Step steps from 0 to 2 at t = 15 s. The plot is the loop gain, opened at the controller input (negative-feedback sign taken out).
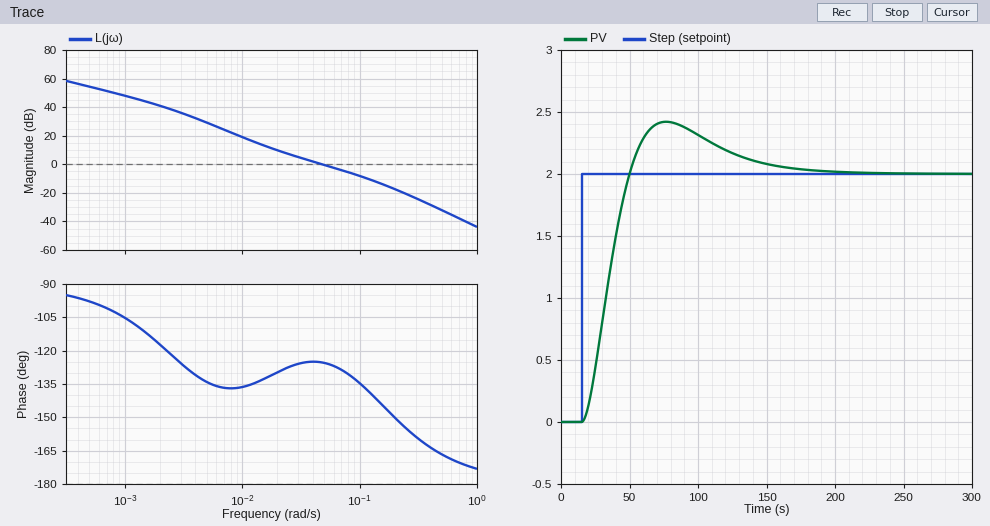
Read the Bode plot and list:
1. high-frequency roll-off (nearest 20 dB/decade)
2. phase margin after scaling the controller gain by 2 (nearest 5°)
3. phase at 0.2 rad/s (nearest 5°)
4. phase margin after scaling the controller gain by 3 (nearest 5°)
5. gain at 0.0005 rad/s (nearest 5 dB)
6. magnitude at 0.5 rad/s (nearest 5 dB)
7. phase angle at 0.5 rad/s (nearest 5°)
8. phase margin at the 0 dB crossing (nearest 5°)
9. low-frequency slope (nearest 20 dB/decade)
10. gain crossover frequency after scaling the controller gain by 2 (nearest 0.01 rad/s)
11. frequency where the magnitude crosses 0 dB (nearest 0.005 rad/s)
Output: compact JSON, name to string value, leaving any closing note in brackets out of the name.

{"high-frequency roll-off": "-40 dB/decade", "phase margin after scaling the controller gain by 2": "50°", "phase at 0.2 rad/s": "-150°", "phase margin after scaling the controller gain by 3": "45°", "gain at 0.0005 rad/s": "55 dB", "magnitude at 0.5 rad/s": "-30 dB", "phase angle at 0.5 rad/s": "-165°", "phase margin at the 0 dB crossing": "55°", "low-frequency slope": "-20 dB/decade", "gain crossover frequency after scaling the controller gain by 2": "0.08 rad/s", "frequency where the magnitude crosses 0 dB": "0.050 rad/s"}
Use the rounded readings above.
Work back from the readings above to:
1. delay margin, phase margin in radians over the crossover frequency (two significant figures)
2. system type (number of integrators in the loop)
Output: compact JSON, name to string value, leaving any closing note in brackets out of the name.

{"delay margin, phase margin in radians over the crossover frequency": "19 s", "system type": "1"}
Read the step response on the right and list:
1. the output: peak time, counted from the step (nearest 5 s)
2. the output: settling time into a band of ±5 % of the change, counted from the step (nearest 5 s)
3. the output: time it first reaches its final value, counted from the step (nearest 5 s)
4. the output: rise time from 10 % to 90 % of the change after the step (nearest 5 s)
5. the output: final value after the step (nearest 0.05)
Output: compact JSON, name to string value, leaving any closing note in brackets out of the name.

{"the output: peak time, counted from the step": "60 s", "the output: settling time into a band of ±5 % of the change, counted from the step": "130 s", "the output: time it first reaches its final value, counted from the step": "35 s", "the output: rise time from 10 % to 90 % of the change after the step": "25 s", "the output: final value after the step": "2.00"}
